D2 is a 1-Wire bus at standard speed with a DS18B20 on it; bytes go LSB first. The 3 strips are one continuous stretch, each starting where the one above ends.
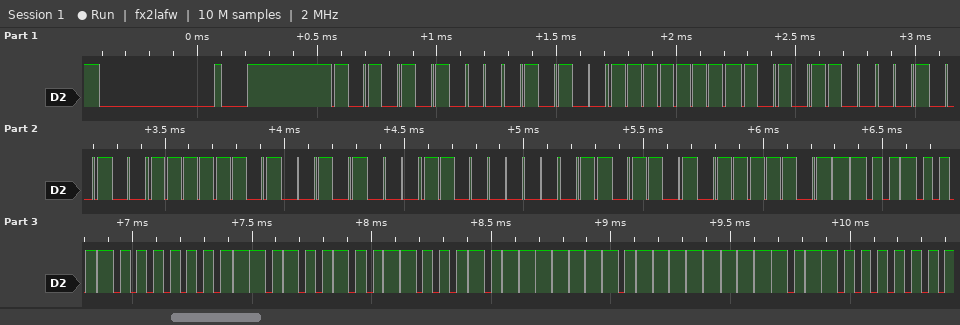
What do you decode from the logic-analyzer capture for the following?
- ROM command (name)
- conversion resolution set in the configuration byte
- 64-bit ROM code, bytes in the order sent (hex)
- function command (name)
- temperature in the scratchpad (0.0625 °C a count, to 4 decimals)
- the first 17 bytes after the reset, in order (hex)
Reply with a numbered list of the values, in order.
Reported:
1. Match ROM
2. 12 bits
3. 28 FF 35 24 BF 14 03 B6
4. Read Scratchpad
5. 17.1875 °C
6. 55 28 FF 35 24 BF 14 03 B6 BE 13 01 4B 46 7F FF 0D
